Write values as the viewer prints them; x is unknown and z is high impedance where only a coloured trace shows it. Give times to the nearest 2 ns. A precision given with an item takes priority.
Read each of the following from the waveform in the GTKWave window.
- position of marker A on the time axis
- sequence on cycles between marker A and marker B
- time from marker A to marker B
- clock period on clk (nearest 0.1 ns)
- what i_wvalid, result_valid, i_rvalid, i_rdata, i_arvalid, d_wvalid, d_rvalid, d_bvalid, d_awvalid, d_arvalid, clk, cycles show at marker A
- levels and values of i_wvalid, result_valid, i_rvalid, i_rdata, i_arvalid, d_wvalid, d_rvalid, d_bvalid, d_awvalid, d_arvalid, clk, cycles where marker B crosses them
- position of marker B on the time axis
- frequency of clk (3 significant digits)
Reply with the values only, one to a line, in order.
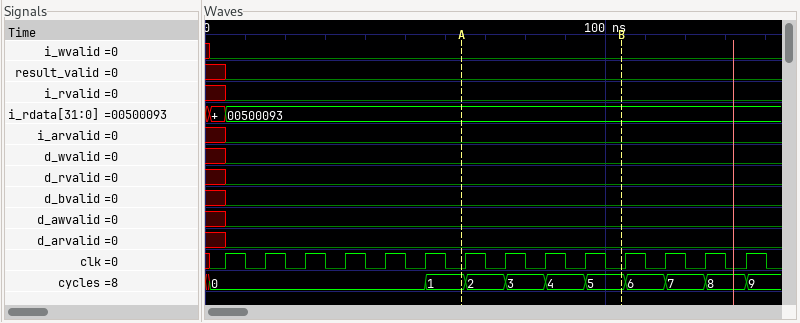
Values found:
64 ns
1, 2, 3, 4, 5
40 ns
10 ns
i_wvalid=0, result_valid=0, i_rvalid=0, i_rdata=00500093, i_arvalid=0, d_wvalid=0, d_rvalid=0, d_bvalid=0, d_awvalid=0, d_arvalid=0, clk=0, cycles=1
i_wvalid=0, result_valid=0, i_rvalid=0, i_rdata=00500093, i_arvalid=0, d_wvalid=0, d_rvalid=0, d_bvalid=0, d_awvalid=0, d_arvalid=0, clk=0, cycles=5
104 ns
100 MHz
